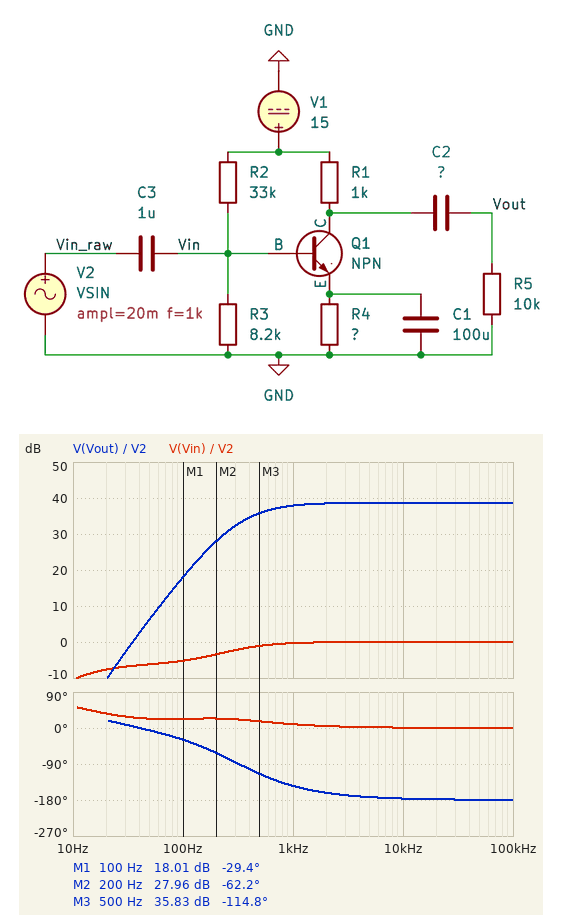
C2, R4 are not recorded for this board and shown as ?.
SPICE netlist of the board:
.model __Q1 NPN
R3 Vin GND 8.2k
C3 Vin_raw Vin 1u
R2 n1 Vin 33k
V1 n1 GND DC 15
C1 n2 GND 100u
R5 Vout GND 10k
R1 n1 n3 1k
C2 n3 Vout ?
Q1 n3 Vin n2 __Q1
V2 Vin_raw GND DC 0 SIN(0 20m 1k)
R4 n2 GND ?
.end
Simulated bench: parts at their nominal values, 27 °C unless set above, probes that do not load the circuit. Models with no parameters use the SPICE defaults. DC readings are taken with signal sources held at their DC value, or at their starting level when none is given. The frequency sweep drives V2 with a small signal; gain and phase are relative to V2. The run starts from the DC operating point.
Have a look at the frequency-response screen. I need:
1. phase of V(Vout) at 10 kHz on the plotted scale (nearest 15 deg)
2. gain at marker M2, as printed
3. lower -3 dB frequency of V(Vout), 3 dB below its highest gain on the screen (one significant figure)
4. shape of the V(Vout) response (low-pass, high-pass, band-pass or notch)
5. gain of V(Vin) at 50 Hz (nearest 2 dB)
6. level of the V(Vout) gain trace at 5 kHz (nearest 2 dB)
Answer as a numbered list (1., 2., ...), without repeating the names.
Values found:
1. -180 deg
2. 27.96 dB
3. 500 Hz
4. high-pass
5. -6 dB
6. 38 dB
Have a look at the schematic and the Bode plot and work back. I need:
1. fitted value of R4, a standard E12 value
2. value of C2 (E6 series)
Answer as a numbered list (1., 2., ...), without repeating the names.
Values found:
1. 820 Ω
2. 47 nF
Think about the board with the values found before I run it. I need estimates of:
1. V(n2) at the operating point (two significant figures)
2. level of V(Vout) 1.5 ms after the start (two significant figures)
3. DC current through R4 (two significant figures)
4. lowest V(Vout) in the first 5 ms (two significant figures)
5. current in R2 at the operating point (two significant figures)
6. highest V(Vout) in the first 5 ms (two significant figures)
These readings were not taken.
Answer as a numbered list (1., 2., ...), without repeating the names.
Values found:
1. 2.0 V
2. 980 mV
3. 2.5 mA
4. -1.8 V
5. 370 µA
6. 1.3 V
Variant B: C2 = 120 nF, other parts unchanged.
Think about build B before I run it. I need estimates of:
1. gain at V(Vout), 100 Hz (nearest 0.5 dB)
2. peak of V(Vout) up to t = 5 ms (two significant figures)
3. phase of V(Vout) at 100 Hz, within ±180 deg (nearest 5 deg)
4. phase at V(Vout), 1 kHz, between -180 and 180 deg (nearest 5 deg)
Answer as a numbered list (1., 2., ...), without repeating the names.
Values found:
1. 24.5 dB
2. 1.4 V
3. -50 deg
4. -155 deg
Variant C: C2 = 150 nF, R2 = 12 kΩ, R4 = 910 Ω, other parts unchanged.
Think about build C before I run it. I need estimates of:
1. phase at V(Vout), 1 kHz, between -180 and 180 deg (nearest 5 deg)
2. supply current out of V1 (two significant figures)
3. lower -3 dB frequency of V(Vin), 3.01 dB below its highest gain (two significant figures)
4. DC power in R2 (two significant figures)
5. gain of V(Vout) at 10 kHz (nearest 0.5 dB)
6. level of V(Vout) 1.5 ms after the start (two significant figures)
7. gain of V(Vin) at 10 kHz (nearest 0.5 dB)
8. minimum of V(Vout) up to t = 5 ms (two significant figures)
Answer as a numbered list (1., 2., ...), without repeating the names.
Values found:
1. -140 deg
2. 6.2 mA
3. 500 Hz
4. 7.0 mW
5. 45.5 dB
6. 1.9 V
7. 0 dB
8. -3.5 V
